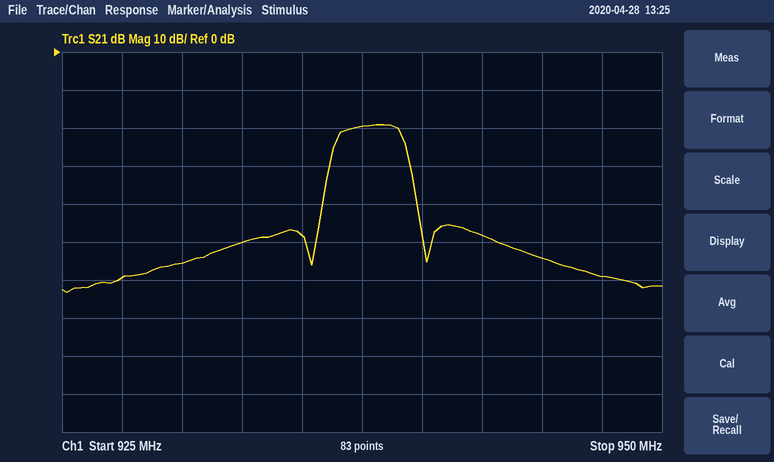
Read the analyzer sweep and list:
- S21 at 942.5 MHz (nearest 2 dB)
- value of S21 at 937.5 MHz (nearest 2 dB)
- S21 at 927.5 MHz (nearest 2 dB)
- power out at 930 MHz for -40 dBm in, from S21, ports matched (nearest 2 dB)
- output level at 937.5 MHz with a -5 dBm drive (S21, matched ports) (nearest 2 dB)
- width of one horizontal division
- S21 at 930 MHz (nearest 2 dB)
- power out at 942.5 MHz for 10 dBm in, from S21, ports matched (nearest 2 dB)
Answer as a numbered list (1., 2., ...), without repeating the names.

1. -48 dB
2. -20 dB
3. -60 dB
4. -96 dBm
5. -24 dBm
6. 2.5 MHz
7. -56 dB
8. -38 dBm
